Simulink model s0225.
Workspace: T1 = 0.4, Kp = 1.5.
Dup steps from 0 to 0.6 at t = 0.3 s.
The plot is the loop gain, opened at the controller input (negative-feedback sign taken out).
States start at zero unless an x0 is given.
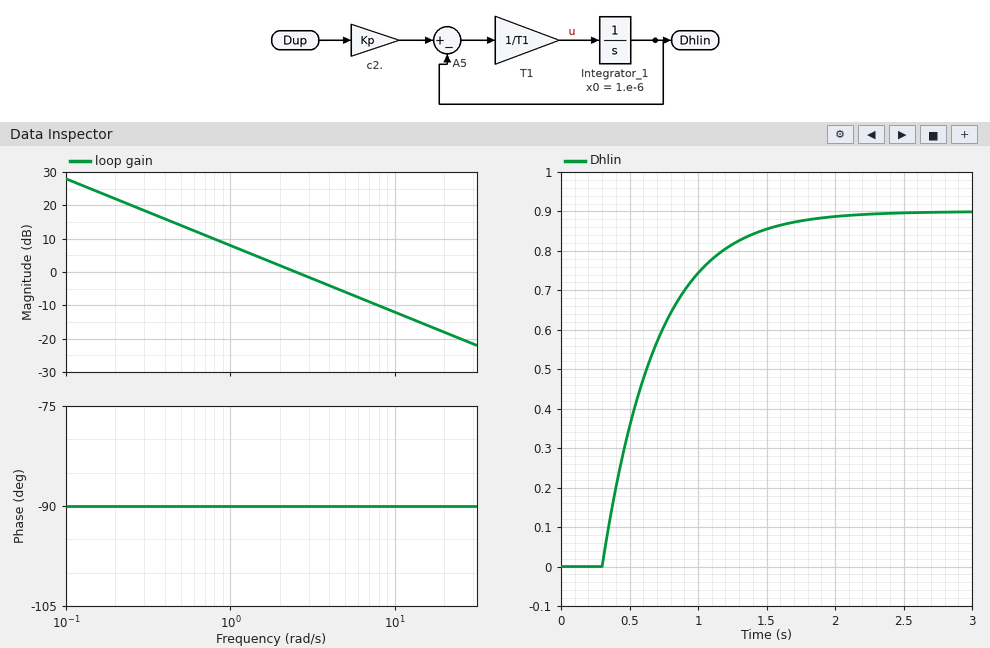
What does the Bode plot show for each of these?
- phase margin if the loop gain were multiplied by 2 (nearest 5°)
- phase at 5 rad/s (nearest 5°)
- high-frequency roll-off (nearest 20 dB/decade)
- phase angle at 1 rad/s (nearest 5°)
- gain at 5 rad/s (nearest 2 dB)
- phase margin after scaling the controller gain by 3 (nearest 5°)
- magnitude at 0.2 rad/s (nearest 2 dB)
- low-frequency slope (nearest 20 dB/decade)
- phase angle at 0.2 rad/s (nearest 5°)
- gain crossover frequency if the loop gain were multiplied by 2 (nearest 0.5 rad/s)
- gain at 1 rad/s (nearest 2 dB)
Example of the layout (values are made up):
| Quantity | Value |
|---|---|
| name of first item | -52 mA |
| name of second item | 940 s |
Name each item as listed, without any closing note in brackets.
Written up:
| Quantity | Value |
|---|---|
| phase margin if the loop gain were multiplied by 2 | 90° |
| phase at 5 rad/s | -90° |
| high-frequency roll-off | -20 dB/decade |
| phase angle at 1 rad/s | -90° |
| gain at 5 rad/s | -6 dB |
| phase margin after scaling the controller gain by 3 | 90° |
| magnitude at 0.2 rad/s | 22 dB |
| low-frequency slope | -20 dB/decade |
| phase angle at 0.2 rad/s | -90° |
| gain crossover frequency if the loop gain were multiplied by 2 | 5.0 rad/s |
| gain at 1 rad/s | 8 dB |
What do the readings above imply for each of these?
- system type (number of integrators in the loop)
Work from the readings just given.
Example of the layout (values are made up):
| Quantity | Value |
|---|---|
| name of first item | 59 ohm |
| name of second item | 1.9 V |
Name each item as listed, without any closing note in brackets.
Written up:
| Quantity | Value |
|---|---|
| system type | 1 |
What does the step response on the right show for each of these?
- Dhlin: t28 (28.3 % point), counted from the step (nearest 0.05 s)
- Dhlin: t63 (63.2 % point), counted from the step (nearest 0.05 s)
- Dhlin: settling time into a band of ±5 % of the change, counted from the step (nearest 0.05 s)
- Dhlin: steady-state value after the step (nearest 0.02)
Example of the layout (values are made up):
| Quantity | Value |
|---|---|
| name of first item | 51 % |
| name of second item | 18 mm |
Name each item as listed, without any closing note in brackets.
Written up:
| Quantity | Value |
|---|---|
| Dhlin: t28 (28.3 % point), counted from the step | 0.15 s |
| Dhlin: t63 (63.2 % point), counted from the step | 0.40 s |
| Dhlin: settling time into a band of ±5 % of the change, counted from the step | 1.20 s |
| Dhlin: steady-state value after the step | 0.90 |
